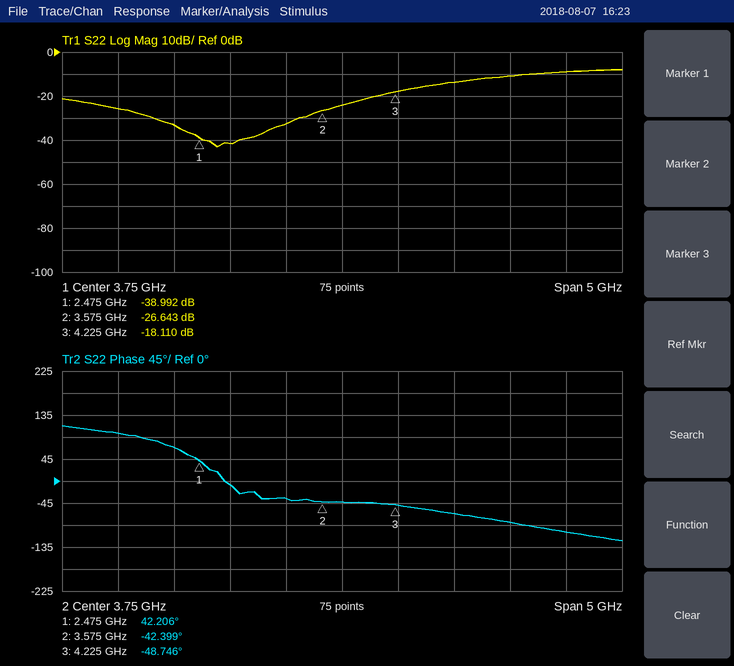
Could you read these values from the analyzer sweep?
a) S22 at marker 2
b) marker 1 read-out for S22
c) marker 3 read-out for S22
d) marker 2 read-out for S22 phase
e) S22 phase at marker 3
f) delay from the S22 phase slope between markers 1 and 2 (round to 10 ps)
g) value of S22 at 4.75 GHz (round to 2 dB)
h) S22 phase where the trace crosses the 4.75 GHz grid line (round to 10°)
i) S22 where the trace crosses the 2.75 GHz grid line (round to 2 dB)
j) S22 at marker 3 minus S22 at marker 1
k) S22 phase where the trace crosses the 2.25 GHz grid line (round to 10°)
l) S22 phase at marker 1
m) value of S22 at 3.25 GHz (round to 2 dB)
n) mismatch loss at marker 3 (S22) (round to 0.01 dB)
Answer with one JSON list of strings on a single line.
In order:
["-26.643 dB", "-38.992 dB", "-18.110 dB", "-42.399°", "-48.746°", "210 ps", "-14 dB", "-70°", "-42 dB", "20.882 dB", "70°", "42.206°", "-32 dB", "0.07 dB"]
